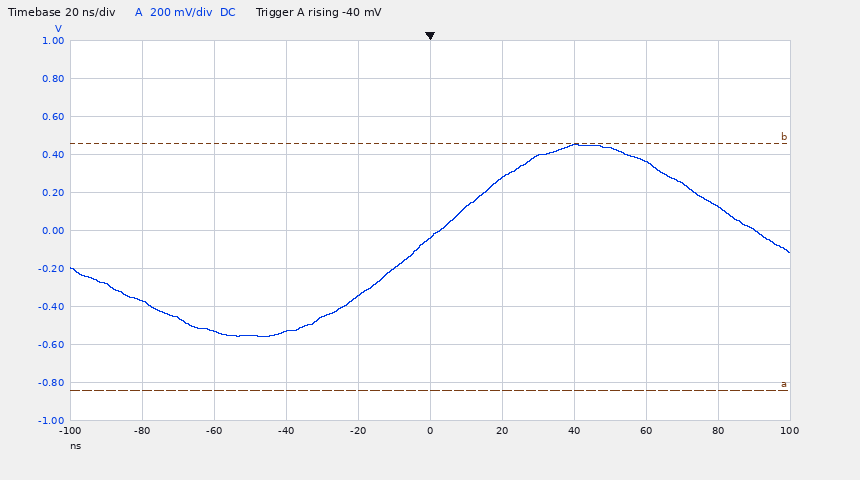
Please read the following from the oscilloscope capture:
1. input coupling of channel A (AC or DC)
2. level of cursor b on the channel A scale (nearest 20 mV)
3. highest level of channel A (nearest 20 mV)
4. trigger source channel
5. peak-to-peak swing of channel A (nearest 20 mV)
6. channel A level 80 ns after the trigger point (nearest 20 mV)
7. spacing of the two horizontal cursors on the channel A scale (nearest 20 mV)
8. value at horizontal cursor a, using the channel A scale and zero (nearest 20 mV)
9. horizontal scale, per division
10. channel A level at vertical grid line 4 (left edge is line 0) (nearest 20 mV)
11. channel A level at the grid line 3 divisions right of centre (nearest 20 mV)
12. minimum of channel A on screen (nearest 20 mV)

DC
460 mV
460 mV
channel A
1.02 V
120 mV
1.30 V
-840 mV
20 ns
-340 mV
360 mV
-560 mV
